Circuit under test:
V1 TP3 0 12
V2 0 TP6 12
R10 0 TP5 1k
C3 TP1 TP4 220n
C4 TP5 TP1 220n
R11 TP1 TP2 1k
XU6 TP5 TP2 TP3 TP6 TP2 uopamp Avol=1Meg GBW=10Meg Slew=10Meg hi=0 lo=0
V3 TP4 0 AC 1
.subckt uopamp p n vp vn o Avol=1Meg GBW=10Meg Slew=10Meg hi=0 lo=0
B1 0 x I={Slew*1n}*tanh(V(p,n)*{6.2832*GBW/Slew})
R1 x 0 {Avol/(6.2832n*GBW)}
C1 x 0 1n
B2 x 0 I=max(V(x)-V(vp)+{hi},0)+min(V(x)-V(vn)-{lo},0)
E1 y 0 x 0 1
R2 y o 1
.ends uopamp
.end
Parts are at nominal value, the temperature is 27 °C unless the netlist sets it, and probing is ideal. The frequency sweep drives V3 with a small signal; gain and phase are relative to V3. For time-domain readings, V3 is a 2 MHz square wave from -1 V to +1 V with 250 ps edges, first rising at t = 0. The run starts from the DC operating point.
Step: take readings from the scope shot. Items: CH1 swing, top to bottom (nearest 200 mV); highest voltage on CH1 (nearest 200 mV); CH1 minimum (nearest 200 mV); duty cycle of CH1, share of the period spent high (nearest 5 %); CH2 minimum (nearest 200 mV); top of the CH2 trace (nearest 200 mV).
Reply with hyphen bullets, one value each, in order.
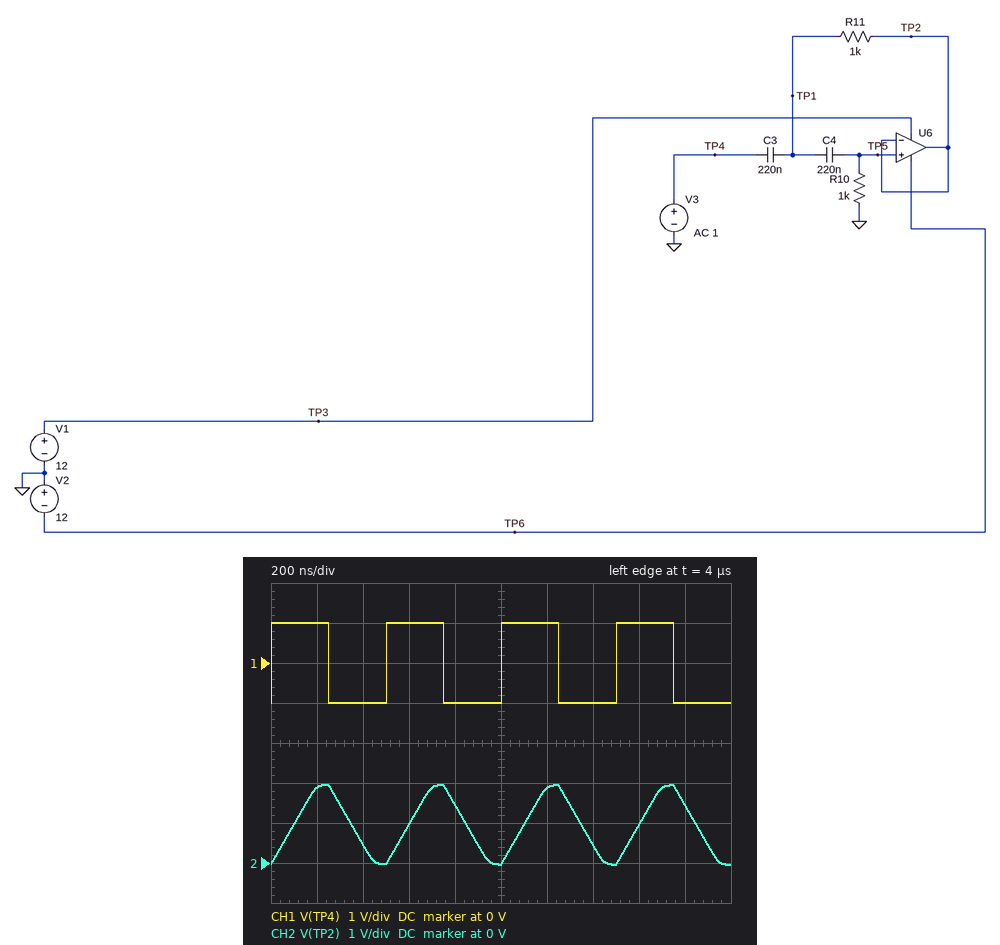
- 2.0 V
- 1.0 V
- -1.0 V
- 50 %
- 0 V
- 2.0 V
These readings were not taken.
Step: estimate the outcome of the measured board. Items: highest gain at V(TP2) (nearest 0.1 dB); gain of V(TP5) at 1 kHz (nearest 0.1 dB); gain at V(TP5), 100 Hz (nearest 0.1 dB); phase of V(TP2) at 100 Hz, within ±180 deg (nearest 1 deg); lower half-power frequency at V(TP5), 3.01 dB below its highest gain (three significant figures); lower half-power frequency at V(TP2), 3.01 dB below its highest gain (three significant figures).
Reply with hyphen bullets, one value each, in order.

- 0 dB
- -3.7 dB
- -34.5 dB
- 164 deg
- 1.12 kHz
- 1.12 kHz
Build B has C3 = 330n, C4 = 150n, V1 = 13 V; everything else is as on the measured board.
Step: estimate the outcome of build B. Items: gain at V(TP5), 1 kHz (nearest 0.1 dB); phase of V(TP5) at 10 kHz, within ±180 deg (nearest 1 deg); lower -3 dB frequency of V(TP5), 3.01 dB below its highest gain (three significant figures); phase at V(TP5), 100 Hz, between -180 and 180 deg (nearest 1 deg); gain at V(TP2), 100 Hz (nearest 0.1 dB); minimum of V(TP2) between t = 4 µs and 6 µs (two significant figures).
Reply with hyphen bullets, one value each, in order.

- -4.2 dB
- 9 deg
- 1.24 kHz
- 163 deg
- -34.4 dB
- -53 mV
